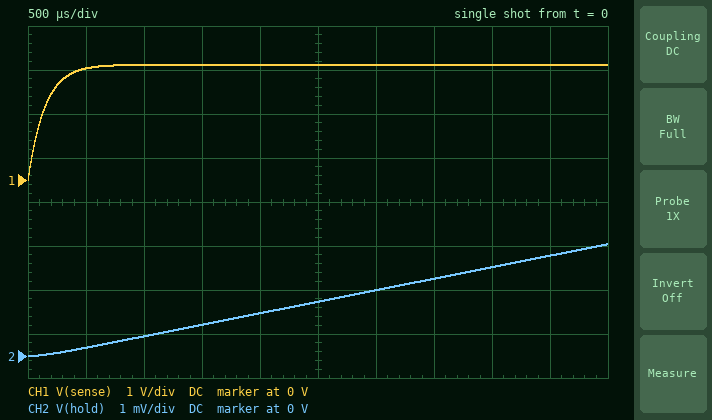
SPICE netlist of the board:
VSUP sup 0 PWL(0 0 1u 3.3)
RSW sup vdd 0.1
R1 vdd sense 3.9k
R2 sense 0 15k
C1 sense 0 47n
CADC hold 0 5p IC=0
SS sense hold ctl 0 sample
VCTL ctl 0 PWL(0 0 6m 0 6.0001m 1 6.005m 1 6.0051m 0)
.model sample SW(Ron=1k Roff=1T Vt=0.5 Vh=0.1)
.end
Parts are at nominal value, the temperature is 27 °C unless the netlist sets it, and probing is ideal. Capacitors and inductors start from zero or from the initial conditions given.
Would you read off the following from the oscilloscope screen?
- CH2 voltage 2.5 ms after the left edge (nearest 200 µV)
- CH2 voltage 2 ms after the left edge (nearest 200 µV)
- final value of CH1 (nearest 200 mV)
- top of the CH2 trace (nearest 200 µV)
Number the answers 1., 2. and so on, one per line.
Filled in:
1. 1.2 mV
2. 1.0 mV
3. 2.6 V
4. 2.6 mV
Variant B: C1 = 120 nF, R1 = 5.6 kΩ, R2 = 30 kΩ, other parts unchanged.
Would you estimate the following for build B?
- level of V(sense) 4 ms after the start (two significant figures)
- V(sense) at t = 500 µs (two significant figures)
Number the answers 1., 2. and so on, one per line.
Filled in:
1. 2.8 V
2. 1.6 V
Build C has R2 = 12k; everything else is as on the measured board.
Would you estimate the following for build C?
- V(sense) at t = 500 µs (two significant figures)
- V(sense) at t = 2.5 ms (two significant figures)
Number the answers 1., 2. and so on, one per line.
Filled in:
1. 2.4 V
2. 2.5 V
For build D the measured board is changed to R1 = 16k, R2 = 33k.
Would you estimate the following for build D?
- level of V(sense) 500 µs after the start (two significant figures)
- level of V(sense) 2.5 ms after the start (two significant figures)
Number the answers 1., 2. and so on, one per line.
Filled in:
1. 1.4 V
2. 2.2 V
